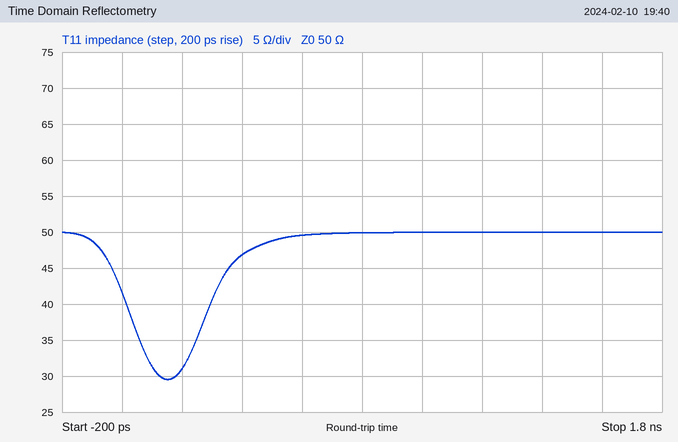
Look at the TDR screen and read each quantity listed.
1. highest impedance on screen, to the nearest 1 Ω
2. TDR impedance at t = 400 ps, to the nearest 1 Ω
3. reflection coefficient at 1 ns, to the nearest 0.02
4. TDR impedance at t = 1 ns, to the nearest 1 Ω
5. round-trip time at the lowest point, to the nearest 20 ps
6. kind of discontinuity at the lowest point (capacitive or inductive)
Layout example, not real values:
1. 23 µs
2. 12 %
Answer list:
1. 50 Ω
2. 47 Ω
3. 0.00
4. 50 Ω
5. 160 ps
6. capacitive
